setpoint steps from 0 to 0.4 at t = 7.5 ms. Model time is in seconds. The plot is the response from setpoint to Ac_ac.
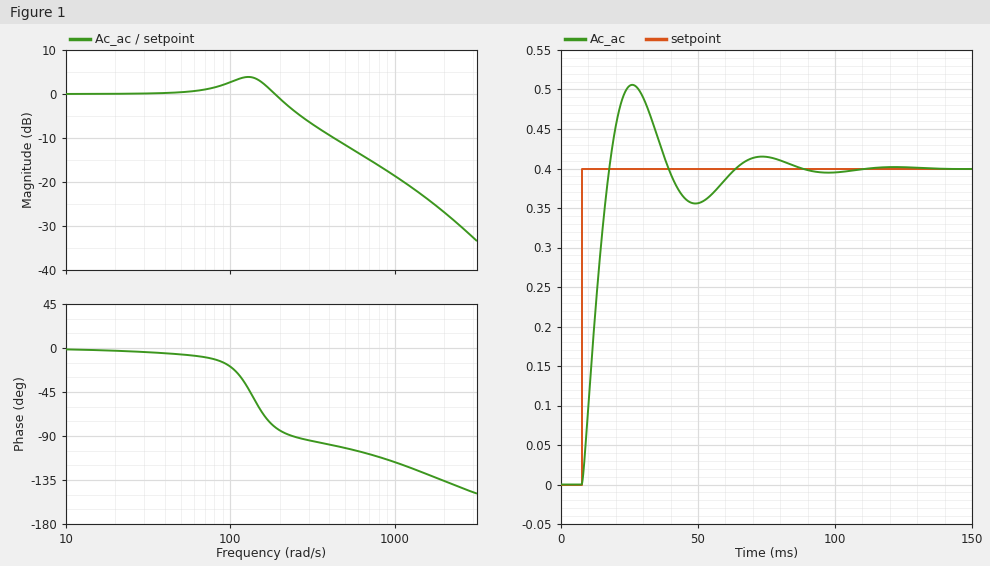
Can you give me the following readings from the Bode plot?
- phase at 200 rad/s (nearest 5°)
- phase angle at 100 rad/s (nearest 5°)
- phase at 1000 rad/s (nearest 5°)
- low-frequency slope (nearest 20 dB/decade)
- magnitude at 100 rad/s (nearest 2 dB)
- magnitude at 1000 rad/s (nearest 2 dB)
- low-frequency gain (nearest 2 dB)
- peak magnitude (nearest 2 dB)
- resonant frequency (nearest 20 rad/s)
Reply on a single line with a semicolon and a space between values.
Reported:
-85°; -20°; -115°; 0 dB/decade; 2 dB; -18 dB; 0 dB; 4 dB; 120 rad/s
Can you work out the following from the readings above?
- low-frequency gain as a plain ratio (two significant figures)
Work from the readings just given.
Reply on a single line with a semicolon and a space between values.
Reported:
1.0
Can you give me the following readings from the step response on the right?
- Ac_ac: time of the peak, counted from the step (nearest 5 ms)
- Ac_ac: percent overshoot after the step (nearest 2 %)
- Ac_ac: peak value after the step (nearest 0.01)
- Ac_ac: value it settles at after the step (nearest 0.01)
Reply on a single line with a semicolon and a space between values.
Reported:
20 ms; 26 %; 0.51; 0.40
